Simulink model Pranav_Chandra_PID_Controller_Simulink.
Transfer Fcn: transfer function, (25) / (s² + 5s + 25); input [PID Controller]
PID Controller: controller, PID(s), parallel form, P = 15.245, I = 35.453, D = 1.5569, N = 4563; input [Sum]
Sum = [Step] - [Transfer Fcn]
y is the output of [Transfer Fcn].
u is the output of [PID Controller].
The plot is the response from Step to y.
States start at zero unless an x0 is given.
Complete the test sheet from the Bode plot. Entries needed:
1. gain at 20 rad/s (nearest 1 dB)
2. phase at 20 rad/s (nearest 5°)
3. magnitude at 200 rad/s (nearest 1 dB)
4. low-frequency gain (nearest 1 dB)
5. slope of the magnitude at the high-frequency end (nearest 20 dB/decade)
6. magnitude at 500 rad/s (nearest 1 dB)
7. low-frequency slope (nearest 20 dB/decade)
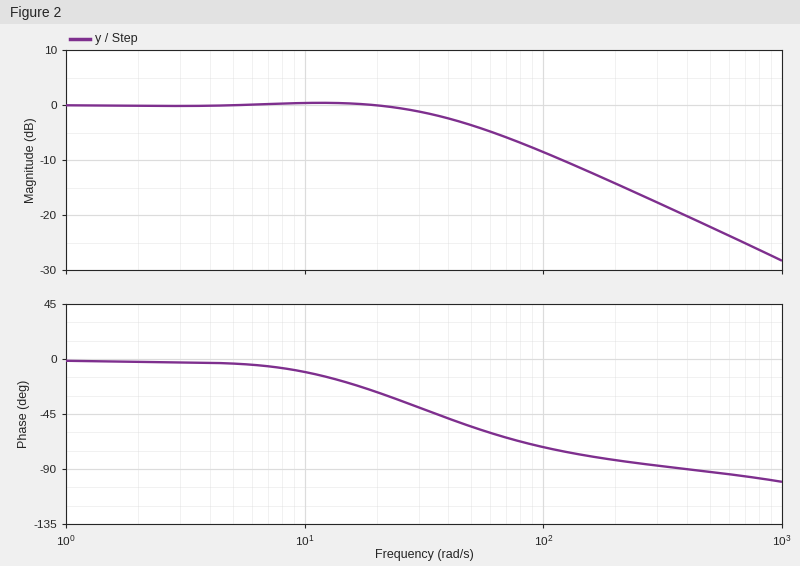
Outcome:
0 dB
-25°
-14 dB
0 dB
-20 dB/decade
-22 dB
0 dB/decade
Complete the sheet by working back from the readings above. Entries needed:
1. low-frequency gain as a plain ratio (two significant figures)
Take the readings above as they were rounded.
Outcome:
1.0
